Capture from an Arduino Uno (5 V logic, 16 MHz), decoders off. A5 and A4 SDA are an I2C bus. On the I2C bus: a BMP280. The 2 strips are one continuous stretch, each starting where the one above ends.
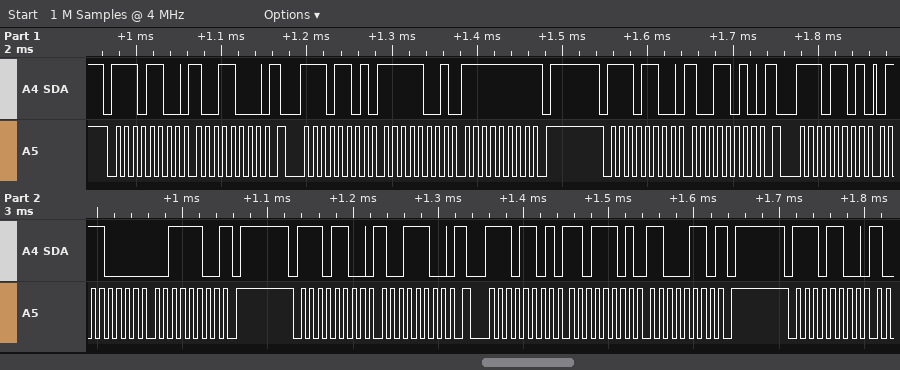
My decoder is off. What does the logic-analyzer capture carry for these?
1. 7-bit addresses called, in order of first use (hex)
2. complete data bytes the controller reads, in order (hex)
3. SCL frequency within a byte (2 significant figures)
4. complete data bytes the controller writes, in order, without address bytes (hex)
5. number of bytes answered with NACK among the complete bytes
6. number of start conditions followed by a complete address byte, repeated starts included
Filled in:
0x76
F9 FF 70 3C DD C6
100 kHz
98 9A 9C
3
7
